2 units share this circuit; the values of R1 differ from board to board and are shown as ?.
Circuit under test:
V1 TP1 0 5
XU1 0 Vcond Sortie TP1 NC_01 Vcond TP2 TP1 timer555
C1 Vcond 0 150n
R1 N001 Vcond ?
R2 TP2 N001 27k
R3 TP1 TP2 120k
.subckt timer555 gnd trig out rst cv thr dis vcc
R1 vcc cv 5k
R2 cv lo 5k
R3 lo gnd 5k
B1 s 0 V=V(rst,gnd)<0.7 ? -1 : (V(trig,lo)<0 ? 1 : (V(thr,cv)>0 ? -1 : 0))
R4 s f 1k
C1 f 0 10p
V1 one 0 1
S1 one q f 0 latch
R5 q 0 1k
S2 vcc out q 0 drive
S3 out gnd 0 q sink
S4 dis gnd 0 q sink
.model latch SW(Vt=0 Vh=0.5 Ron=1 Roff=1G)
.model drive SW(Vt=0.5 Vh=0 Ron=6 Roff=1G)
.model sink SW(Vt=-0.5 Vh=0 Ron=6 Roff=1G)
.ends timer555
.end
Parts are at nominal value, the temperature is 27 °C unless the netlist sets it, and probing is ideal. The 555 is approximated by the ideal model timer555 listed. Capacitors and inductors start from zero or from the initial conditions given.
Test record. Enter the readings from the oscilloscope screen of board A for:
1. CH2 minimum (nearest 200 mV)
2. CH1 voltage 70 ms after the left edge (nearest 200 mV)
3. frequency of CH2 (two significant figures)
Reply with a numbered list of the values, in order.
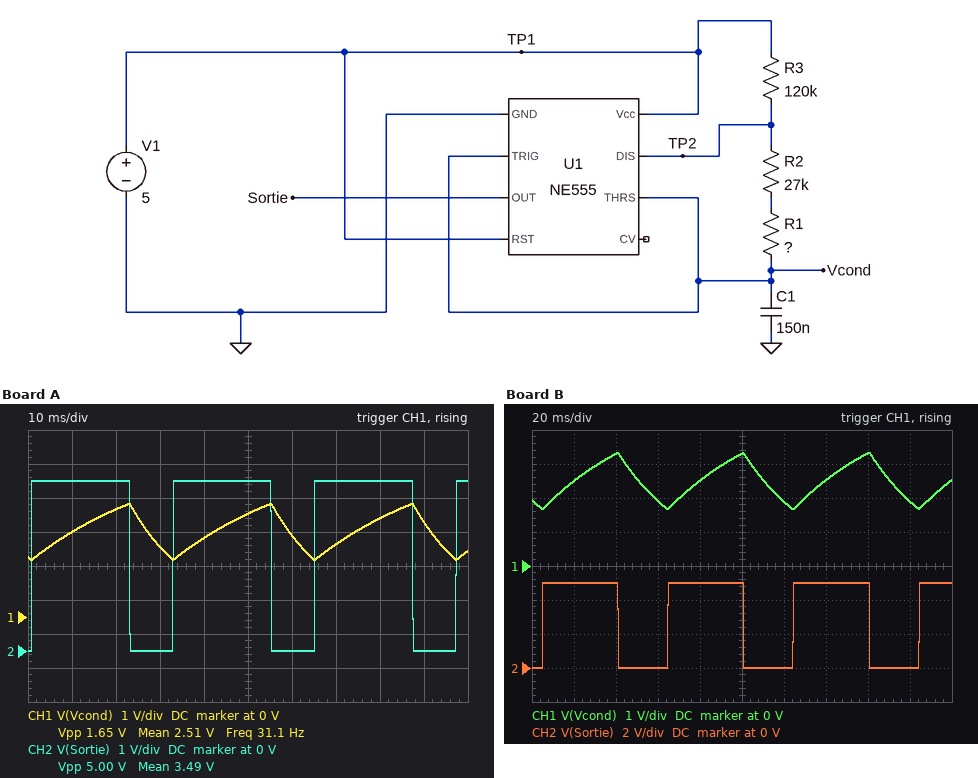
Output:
1. 0 V
2. 2.2 V
3. 31 Hz
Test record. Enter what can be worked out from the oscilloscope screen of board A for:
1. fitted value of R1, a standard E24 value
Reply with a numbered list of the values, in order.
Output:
1. 68 kΩ
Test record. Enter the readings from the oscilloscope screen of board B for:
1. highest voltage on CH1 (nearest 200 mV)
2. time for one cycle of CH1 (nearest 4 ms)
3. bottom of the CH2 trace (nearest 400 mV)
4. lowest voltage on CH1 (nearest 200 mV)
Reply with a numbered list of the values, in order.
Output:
1. 3.4 V
2. 60 ms
3. 0 V
4. 1.6 V
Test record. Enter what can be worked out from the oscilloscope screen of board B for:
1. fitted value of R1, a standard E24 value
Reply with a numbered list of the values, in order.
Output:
1. 200 kΩ
